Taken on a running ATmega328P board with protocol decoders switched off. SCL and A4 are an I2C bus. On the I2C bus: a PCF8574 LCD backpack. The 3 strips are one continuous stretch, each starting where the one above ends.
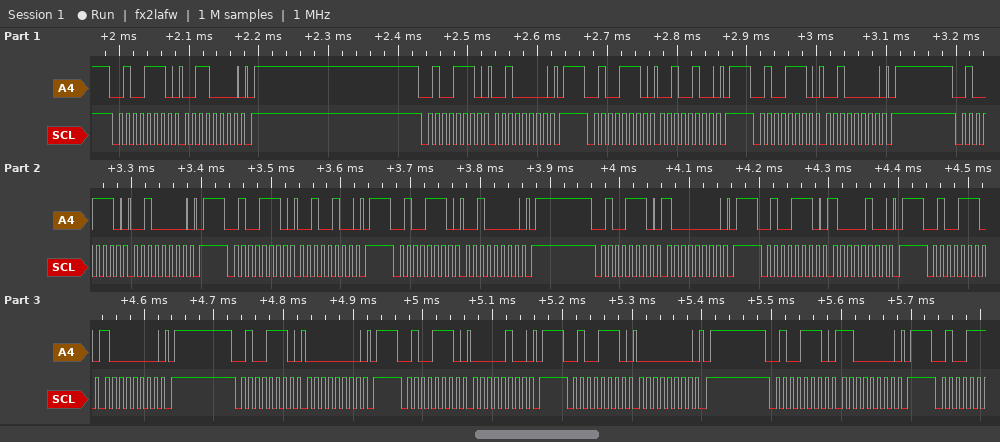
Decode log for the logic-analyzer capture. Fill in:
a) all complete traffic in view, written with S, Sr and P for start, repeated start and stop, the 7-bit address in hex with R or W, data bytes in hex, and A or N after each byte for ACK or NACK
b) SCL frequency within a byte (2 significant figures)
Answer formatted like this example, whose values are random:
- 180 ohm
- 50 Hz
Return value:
- S 27W A 30 A P S 27W A 20 A P S 27W A 24 A P S 27W A 20 A P S 27W A 20 A P S 27W A 24 A P S 27W A 20 A P S 27W A 80 A P S 27W A 84 A P S 27W A 80 A P S 27W A 00 A P S 27W A 04 A P S 27W A 00 A P S 27W A C0 A P
- 100 kHz
